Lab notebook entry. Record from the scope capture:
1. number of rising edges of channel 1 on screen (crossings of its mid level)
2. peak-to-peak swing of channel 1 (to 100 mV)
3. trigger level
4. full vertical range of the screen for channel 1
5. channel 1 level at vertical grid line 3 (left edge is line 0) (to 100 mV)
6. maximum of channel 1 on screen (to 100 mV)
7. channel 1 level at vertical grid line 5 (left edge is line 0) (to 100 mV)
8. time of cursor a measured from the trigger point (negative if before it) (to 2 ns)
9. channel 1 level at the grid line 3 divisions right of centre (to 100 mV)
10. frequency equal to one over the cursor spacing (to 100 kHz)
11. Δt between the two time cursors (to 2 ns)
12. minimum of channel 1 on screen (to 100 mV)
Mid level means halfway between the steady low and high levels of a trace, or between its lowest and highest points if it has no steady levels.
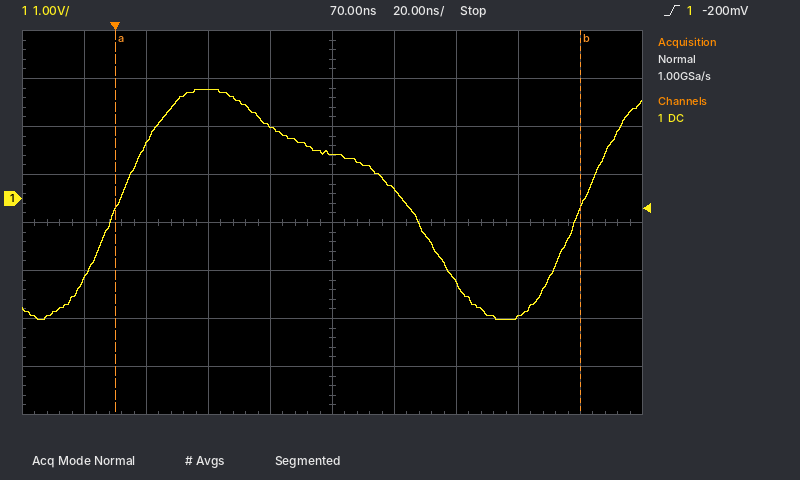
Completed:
2
4.8 V
-200 mV
8 V
2.3 V
2.3 V
900 mV
0 ns
-2.5 V
6.7 MHz
150 ns
-2.5 V
